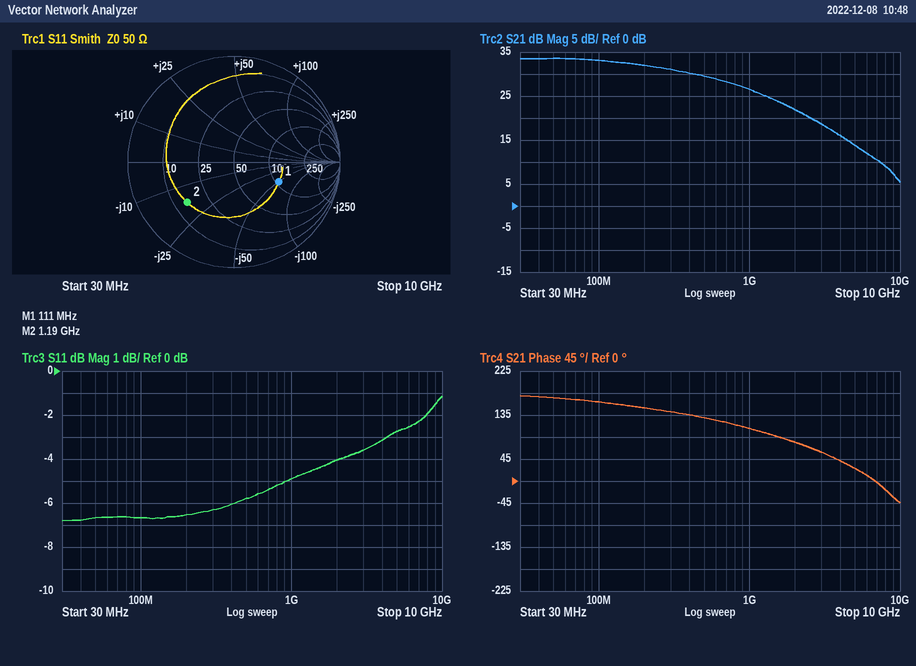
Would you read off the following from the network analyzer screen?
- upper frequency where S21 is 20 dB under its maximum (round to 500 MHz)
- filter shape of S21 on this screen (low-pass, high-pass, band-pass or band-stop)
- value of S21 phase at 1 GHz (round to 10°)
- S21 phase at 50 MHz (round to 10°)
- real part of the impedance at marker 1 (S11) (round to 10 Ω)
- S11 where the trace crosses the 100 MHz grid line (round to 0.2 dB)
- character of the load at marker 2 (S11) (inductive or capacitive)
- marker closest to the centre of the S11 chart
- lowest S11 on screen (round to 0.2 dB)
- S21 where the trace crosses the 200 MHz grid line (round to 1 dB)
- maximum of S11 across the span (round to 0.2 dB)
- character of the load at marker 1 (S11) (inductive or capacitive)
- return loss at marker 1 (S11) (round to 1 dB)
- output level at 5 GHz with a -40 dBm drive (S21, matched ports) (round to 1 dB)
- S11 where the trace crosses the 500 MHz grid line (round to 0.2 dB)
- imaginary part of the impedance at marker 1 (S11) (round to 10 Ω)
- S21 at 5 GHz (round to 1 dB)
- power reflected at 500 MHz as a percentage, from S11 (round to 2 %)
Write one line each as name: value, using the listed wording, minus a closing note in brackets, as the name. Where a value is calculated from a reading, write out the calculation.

upper frequency where S21 is 20 dB under its maximum: 5.0 GHz
filter shape of S21 on this screen: low-pass
value of S21 phase at 1 GHz: 110°
S21 phase at 50 MHz: 170°
real part of the impedance at marker 1 (S11): 110 Ω
S11 where the trace crosses the 100 MHz grid line: -6.6 dB
character of the load at marker 2 (S11): capacitive
marker closest to the centre of the S11 chart: marker 1
lowest S11 on screen: -6.8 dB
S21 where the trace crosses the 200 MHz grid line: 32 dB
maximum of S11 across the span: -1.2 dB
character of the load at marker 1 (S11): capacitive
return loss at marker 1 (S11): 7 dB
output level at 5 GHz with a -40 dBm drive (S21, matched ports): -40 dBm + (14 dB) = -26 dBm
S11 where the trace crosses the 500 MHz grid line: -5.8 dB
imaginary part of the impedance at marker 1 (S11): -50 Ω
S21 at 5 GHz: 14 dB
power reflected at 500 MHz as a percentage, from S11: 10^(-5.8/10) ≈ 26 %
